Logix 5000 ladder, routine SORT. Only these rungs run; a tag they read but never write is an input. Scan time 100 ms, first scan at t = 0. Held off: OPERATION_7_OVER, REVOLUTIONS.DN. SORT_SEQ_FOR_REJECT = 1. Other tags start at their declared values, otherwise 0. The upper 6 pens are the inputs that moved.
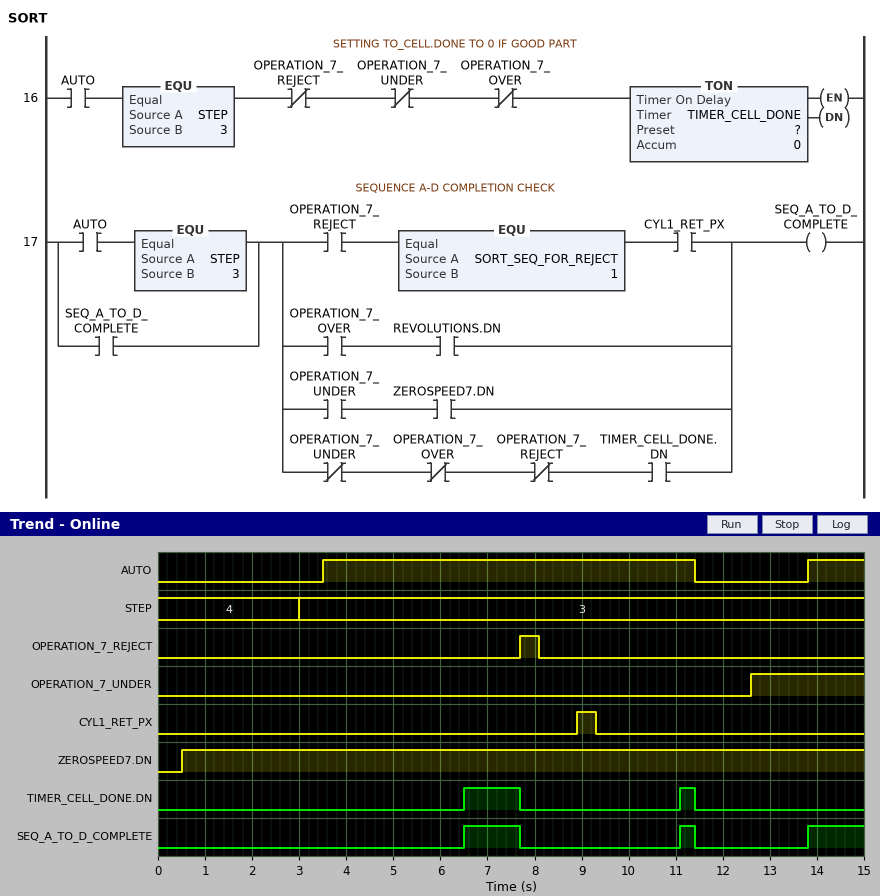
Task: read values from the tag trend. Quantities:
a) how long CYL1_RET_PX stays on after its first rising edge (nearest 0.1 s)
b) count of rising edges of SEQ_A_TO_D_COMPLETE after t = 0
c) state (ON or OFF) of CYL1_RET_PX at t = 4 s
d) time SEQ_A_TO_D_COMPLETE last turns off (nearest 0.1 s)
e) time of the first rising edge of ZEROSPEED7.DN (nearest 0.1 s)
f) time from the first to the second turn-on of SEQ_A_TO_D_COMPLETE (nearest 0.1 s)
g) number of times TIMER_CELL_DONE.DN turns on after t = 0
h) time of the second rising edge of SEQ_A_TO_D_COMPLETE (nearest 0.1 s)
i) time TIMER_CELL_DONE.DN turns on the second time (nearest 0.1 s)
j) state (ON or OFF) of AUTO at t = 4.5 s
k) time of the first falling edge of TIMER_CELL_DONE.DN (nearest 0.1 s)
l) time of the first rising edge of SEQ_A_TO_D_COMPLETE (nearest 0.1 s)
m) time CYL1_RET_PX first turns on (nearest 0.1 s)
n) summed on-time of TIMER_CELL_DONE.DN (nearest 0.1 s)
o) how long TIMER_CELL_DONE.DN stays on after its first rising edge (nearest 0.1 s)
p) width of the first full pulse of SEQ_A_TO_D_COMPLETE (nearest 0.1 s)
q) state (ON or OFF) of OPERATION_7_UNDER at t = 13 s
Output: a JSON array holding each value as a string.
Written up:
["0.4 s", "3", "OFF", "11.4 s", "0.5 s", "4.6 s", "2", "11.1 s", "11.1 s", "ON", "7.7 s", "6.5 s", "8.9 s", "1.5 s", "1.2 s", "1.2 s", "ON"]
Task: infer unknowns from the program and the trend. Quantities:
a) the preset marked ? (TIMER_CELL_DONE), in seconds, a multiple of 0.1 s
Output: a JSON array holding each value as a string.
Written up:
["3.0 s"]
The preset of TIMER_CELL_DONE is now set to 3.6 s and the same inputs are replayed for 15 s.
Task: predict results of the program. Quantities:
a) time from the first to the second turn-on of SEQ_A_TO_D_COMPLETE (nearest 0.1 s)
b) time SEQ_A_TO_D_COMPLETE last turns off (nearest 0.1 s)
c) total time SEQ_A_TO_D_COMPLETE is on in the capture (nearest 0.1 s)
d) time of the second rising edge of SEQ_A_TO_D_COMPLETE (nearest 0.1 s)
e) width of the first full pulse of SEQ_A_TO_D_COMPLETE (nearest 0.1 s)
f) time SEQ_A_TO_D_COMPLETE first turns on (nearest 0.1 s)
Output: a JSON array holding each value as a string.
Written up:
["6.7 s", "7.7 s", "1.8 s", "13.8 s", "0.6 s", "7.1 s"]
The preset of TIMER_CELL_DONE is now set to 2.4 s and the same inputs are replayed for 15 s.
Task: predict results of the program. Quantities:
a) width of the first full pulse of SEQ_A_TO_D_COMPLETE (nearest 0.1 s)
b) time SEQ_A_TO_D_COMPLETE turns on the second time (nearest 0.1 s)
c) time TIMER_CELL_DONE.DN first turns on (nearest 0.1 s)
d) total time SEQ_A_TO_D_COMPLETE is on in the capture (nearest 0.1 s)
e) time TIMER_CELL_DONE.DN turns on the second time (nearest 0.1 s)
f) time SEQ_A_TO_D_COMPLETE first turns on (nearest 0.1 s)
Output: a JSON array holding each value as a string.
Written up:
["1.8 s", "10.5 s", "5.9 s", "3.9 s", "10.5 s", "5.9 s"]
